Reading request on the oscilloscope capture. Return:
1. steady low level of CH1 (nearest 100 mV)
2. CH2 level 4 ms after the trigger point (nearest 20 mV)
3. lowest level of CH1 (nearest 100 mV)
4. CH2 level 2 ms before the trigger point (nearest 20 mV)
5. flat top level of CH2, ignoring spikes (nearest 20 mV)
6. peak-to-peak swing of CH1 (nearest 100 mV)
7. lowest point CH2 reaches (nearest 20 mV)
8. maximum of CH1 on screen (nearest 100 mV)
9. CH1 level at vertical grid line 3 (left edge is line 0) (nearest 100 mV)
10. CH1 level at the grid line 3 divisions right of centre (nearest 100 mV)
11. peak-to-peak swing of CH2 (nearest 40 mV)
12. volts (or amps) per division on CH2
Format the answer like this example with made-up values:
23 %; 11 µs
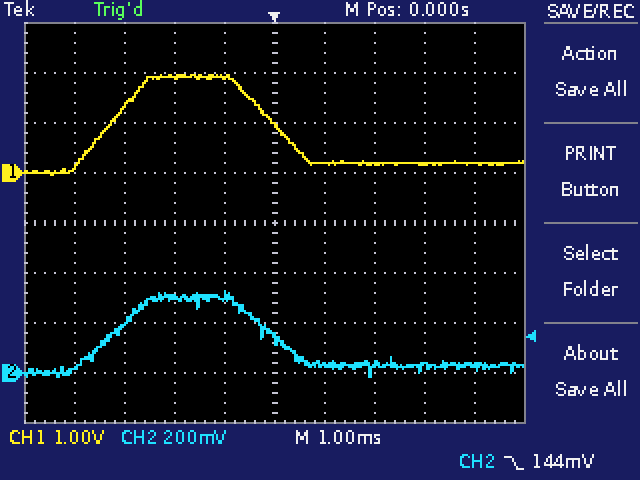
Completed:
200 mV; 20 mV; 0.0 V; 300 mV; 300 mV; 2.0 V; -20 mV; 2.0 V; 1.9 V; 200 mV; 360 mV; 200 mV
